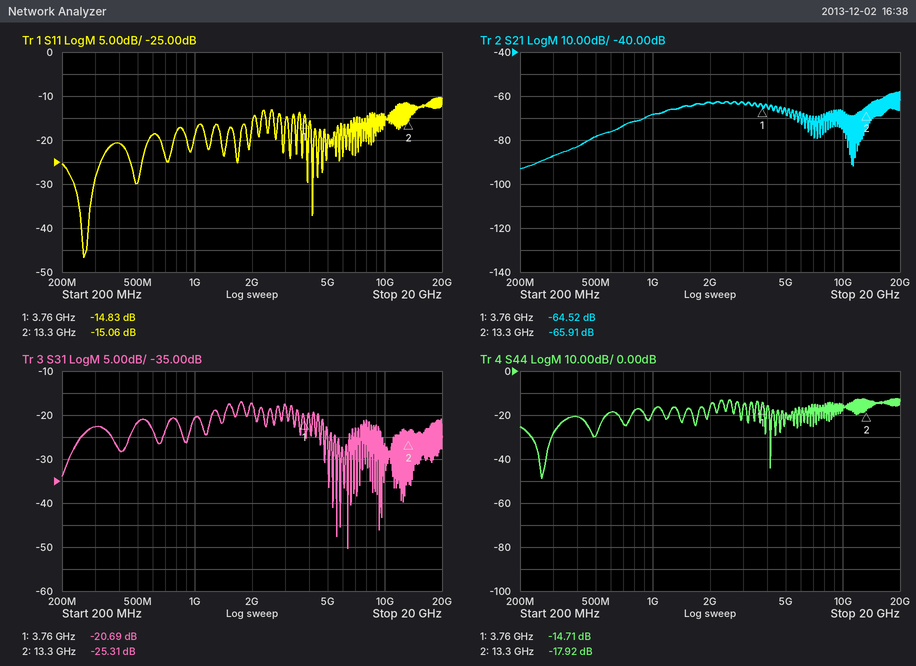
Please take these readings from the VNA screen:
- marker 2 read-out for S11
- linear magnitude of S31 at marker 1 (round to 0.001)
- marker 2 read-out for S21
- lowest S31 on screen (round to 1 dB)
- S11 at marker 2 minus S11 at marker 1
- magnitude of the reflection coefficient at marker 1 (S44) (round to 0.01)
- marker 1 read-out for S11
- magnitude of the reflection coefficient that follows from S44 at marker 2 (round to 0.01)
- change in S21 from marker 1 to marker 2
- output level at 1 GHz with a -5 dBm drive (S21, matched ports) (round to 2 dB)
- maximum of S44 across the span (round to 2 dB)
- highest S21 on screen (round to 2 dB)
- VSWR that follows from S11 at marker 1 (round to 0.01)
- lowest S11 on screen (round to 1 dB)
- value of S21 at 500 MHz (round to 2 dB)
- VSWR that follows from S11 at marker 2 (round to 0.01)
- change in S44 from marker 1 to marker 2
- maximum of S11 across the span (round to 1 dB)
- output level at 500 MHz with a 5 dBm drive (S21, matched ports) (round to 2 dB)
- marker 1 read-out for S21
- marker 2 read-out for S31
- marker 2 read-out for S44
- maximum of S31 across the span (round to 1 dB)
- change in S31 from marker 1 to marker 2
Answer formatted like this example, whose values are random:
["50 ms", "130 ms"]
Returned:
["-15.06 dB", "0.092", "-65.91 dB", "-50 dB", "-0.23 dB", "0.18", "-14.83 dB", "0.13", "-1.39 dB", "-74 dBm", "-12 dB", "-58 dB", "1.44", "-47 dB", "-78 dB", "1.43", "-3.21 dB", "-10 dB", "-74 dBm", "-64.52 dB", "-25.31 dB", "-17.92 dB", "-17 dB", "-4.62 dB"]
